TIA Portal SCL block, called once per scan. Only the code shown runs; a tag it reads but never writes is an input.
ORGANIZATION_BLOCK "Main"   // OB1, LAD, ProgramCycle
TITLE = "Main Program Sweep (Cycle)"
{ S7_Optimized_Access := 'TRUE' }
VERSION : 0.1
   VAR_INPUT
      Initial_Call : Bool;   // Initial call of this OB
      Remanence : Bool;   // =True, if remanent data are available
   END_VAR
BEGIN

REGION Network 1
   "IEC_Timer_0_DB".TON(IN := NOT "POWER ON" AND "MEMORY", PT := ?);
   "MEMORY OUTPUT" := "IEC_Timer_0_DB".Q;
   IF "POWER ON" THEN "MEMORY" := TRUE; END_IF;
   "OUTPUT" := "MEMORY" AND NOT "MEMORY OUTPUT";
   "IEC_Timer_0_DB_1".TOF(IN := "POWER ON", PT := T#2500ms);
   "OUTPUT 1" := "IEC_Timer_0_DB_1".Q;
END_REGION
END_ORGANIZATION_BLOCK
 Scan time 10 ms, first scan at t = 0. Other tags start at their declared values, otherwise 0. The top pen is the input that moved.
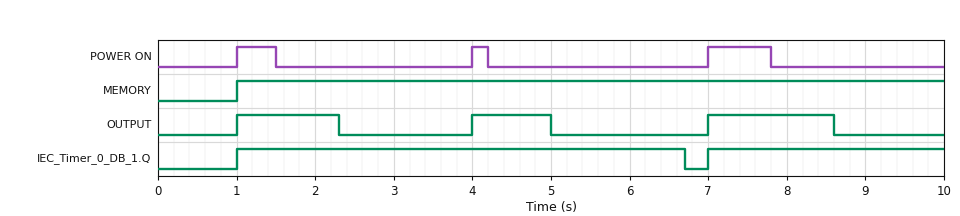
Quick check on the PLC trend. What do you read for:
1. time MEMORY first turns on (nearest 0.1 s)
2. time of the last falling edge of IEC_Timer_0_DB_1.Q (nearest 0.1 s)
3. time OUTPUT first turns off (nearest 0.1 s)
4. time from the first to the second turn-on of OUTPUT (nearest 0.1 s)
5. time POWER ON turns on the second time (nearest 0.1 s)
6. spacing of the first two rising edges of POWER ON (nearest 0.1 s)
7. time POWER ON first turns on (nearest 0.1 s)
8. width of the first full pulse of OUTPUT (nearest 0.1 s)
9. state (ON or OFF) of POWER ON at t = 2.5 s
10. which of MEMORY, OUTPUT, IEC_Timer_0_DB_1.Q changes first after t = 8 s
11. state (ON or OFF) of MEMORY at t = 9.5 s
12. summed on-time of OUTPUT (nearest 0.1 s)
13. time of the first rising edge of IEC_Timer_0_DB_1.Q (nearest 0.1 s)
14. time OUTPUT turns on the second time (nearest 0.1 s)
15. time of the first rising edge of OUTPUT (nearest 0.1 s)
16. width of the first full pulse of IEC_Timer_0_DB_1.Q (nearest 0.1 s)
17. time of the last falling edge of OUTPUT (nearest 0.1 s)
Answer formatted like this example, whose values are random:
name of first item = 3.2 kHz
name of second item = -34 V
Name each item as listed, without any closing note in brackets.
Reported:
time MEMORY first turns on = 1.0 s
time of the last falling edge of IEC_Timer_0_DB_1.Q = 6.7 s
time OUTPUT first turns off = 2.3 s
time from the first to the second turn-on of OUTPUT = 3.0 s
time POWER ON turns on the second time = 4.0 s
spacing of the first two rising edges of POWER ON = 3.0 s
time POWER ON first turns on = 1.0 s
width of the first full pulse of OUTPUT = 1.3 s
state (ON or OFF) of POWER ON at t = 2.5 s = OFF
which of MEMORY, OUTPUT, IEC_Timer_0_DB_1.Q changes first after t = 8 s = OUTPUT
state (ON or OFF) of MEMORY at t = 9.5 s = ON
summed on-time of OUTPUT = 3.9 s
time of the first rising edge of IEC_Timer_0_DB_1.Q = 1.0 s
time OUTPUT turns on the second time = 4.0 s
time of the first rising edge of OUTPUT = 1.0 s
width of the first full pulse of IEC_Timer_0_DB_1.Q = 5.7 s
time of the last falling edge of OUTPUT = 8.6 s
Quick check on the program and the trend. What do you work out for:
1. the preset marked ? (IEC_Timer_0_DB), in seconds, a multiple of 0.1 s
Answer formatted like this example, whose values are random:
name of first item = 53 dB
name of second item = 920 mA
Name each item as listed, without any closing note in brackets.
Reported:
the preset marked ? (IEC_Timer_0_DB), in seconds, a multiple of 0.1 s = 0.8 s
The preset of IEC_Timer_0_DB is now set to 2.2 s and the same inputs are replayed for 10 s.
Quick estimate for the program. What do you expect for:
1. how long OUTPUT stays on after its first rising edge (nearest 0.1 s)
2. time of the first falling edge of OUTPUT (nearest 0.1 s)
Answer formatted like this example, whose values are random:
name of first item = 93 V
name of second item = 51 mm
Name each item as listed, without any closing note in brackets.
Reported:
how long OUTPUT stays on after its first rising edge = 2.7 s
time of the first falling edge of OUTPUT = 3.7 s
